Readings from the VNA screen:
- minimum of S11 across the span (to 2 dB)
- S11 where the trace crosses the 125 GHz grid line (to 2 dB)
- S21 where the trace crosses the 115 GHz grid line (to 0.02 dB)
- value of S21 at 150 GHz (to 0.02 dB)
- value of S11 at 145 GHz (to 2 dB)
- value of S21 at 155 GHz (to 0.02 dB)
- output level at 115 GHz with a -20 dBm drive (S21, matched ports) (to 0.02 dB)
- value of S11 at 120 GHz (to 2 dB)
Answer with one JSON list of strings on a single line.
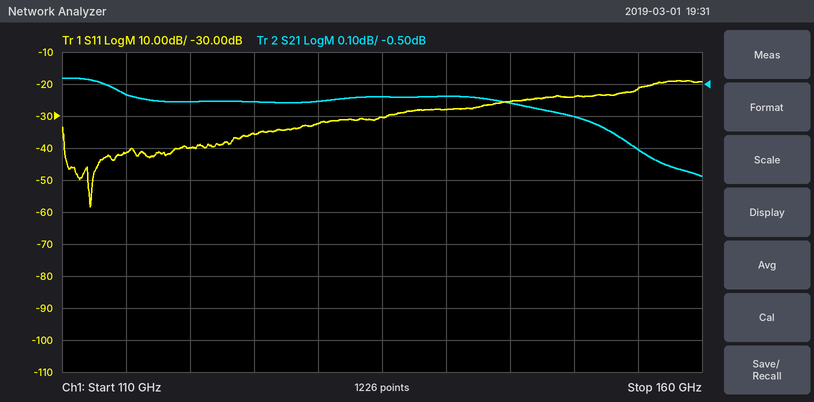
["-58 dB", "-36 dB", "-0.54 dB", "-0.60 dB", "-26 dB", "-0.70 dB", "-20.54 dBm", "-40 dB"]
